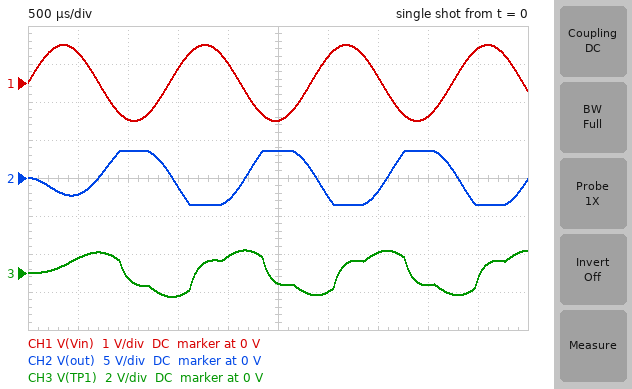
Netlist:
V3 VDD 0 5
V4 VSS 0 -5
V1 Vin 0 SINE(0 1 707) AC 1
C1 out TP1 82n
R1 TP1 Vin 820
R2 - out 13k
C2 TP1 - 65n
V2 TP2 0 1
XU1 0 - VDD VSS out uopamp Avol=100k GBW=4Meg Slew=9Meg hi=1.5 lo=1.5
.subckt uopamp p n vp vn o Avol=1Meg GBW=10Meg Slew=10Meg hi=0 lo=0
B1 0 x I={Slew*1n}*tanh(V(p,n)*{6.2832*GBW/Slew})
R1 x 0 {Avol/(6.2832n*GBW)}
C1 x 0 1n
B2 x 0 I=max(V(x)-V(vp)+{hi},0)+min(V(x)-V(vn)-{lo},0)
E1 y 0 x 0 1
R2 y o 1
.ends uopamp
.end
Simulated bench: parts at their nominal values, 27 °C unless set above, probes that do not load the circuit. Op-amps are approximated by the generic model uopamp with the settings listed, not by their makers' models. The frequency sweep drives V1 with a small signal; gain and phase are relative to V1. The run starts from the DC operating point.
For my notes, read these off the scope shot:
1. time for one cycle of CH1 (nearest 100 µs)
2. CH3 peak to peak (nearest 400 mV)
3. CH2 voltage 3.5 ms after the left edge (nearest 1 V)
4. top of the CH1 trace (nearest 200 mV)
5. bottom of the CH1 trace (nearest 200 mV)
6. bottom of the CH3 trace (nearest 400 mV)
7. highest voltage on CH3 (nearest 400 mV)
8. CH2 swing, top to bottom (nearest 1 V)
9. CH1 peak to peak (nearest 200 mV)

1.4 ms
2.4 V
-2 V
1.0 V
-1.0 V
-1.2 V
1.2 V
7 V
2.0 V
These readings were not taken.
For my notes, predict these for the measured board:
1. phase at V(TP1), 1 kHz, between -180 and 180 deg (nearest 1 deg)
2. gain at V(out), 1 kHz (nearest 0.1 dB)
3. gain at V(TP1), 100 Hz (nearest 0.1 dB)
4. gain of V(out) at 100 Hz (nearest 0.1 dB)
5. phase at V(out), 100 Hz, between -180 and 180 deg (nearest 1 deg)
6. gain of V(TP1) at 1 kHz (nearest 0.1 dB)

-149 deg
11.2 dB
0.2 dB
-5.3 dB
-94 deg
-3.3 dB
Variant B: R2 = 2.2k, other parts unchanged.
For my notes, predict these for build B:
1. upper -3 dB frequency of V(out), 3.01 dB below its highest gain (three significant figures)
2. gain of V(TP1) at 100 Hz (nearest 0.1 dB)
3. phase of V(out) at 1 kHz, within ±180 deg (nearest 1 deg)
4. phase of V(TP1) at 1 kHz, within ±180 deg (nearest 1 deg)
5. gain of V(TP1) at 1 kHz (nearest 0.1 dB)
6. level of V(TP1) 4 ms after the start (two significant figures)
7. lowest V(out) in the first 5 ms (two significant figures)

2.90 kHz
0 dB
-141 deg
-51 deg
0.2 dB
-1.0 V
-650 mV
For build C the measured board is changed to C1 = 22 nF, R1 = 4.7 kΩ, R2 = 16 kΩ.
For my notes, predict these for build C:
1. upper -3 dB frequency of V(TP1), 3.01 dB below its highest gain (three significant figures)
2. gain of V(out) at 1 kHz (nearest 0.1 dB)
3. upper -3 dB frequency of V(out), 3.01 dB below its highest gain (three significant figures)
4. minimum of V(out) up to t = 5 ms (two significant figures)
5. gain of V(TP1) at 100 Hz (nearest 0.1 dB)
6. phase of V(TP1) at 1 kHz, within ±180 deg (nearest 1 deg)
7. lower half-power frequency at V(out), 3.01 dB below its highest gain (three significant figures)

531 Hz
4.0 dB
874 Hz
-2.2 V
0.1 dB
-142 deg
269 Hz
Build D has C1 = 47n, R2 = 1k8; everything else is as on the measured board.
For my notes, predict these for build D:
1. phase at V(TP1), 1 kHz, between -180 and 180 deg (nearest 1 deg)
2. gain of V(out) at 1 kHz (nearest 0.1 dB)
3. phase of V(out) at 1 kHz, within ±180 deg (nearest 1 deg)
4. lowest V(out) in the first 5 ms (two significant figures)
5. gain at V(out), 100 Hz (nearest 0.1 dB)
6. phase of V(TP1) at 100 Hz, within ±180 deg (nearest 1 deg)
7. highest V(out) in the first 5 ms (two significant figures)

-35 deg
-2.7 dB
-125 deg
-520 mV
-22.7 dB
-3 deg
520 mV
